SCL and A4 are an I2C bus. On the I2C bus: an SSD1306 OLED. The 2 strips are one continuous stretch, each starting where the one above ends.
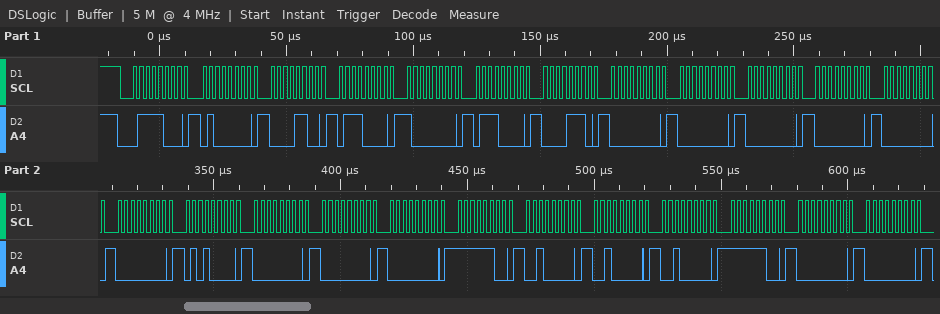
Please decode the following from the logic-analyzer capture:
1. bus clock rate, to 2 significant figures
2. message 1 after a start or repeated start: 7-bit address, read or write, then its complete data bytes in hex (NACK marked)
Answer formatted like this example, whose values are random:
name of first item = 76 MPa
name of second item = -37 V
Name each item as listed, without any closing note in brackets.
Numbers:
bus clock rate, to 2 significant figures = 400 kHz
message 1 after a start or repeated start: 7-bit address, read or write, then its complete data bytes in hex = 0x3C write: 40 0C 70 80 70 0E 00 00 00 00 00 00 50 00 00 00 FC 20 20 20 FC 00 00
